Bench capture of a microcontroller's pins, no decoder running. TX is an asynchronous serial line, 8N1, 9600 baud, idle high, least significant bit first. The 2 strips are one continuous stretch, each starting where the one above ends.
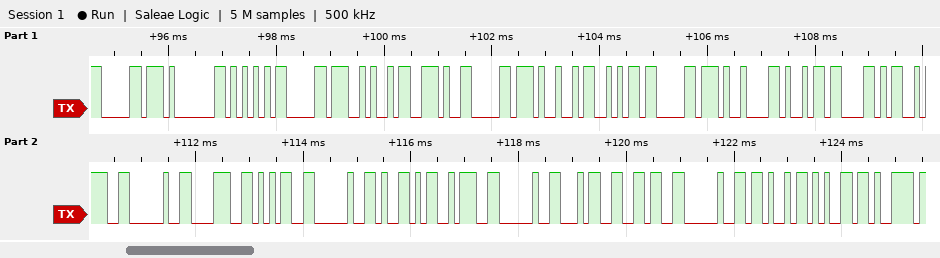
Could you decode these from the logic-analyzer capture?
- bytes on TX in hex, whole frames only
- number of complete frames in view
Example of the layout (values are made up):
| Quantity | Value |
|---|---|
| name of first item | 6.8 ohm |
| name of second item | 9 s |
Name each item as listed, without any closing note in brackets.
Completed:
| Quantity | Value |
|---|---|
| bytes on TX in hex, whole frames only | 0xB0 0x01 0x55 0xB0 0x4A 0x2E 0xB0 0x49 0x6A 0xB0 0x09 0x69 0x58 0x3A 0x20 0x38 0x35 0x20 0x59 0x3A 0x20 0x34 0x36 0x20 0x4B 0x65 0x79 |
| number of complete frames in view | 27 |
